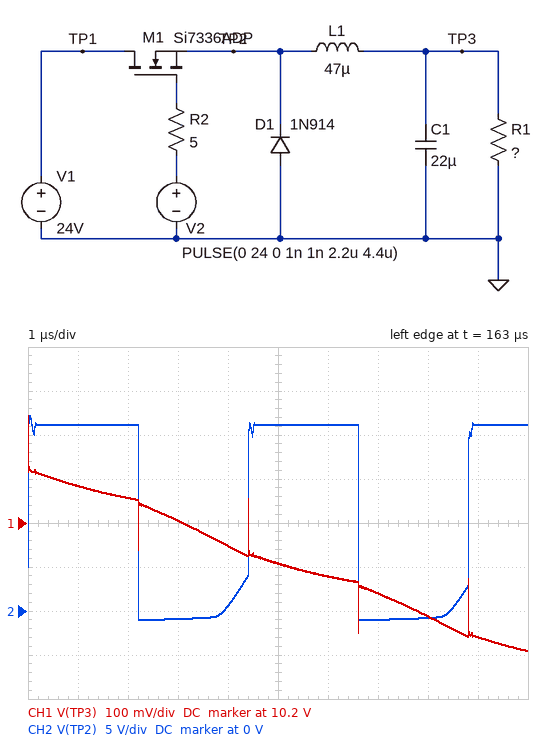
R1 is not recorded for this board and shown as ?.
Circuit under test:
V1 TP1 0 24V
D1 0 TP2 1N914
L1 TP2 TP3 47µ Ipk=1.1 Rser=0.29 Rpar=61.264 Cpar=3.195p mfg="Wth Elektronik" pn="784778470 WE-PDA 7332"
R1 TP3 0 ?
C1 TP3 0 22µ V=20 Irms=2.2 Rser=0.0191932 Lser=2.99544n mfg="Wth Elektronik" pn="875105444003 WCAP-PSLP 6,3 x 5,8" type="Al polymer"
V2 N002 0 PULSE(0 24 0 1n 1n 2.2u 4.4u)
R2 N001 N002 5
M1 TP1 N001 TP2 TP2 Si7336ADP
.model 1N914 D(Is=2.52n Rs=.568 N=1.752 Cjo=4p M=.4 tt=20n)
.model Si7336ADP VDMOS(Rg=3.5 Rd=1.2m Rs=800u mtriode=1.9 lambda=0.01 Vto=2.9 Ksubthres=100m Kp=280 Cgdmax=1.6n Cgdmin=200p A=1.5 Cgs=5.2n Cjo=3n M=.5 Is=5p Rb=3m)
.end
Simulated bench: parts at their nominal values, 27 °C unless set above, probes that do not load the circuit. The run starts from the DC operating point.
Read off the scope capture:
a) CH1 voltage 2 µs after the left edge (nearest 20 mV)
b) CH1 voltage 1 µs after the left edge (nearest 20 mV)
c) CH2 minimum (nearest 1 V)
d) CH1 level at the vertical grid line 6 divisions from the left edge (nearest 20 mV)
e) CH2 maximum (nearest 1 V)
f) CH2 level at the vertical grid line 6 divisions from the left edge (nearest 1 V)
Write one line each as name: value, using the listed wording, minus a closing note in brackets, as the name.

CH1 voltage 2 µs after the left edge: 10.26 V
CH1 voltage 1 µs after the left edge: 10.28 V
CH2 minimum: -1 V
CH1 level at the vertical grid line 6 divisions from the left edge: 10.08 V
CH2 maximum: 22 V
CH2 level at the vertical grid line 6 divisions from the left edge: 21 V
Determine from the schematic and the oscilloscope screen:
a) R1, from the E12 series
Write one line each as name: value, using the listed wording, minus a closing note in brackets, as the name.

R1, from the E12 series: 8.2 Ω
